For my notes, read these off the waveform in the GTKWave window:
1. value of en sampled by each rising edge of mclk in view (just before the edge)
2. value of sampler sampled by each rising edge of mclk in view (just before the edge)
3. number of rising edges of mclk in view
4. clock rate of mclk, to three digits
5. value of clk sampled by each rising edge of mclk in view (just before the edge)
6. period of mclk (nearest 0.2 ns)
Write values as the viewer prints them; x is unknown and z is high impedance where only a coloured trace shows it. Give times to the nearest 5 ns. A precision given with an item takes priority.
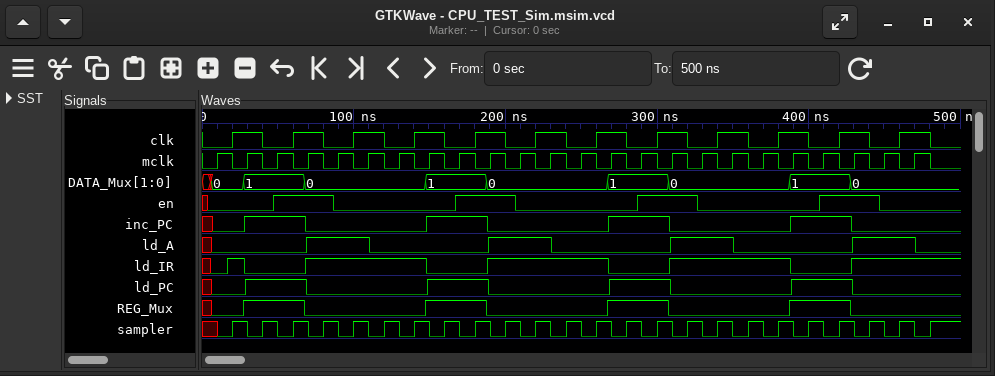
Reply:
0 0 1 1 0 0 0 0 1 1 0 0 0 0 1 1 0 0 0 0 1 1 0 0
x 1 1 1 1 1 1 1 1 1 1 1 1 1 1 1 1 1 1 1 1 1 1 1
24
50.0 MHz
0 1 0 1 0 1 0 1 0 1 0 1 0 1 0 1 0 1 0 1 0 1 0 1
20 ns
